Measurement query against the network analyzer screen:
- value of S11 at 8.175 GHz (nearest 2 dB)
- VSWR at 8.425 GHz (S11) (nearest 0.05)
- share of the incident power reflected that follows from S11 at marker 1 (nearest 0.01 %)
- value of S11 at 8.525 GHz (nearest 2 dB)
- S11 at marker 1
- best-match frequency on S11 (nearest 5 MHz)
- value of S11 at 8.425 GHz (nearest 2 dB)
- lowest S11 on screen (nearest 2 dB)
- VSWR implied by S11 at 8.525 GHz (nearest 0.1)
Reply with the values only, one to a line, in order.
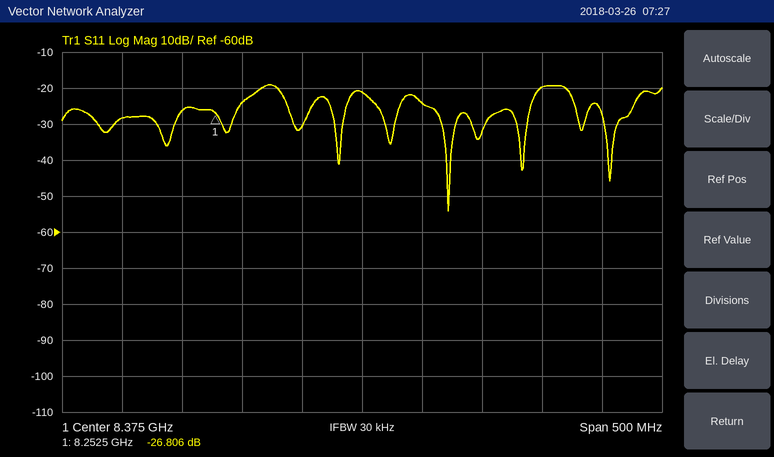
-28 dB
1.15
0.21 %
-20 dB
-26.806 dB
8.445 GHz
-24 dB
-54 dB
1.2
